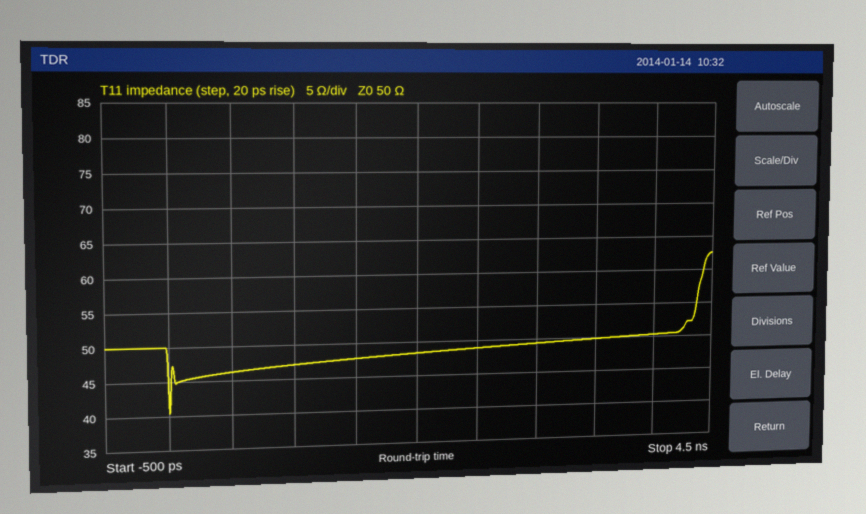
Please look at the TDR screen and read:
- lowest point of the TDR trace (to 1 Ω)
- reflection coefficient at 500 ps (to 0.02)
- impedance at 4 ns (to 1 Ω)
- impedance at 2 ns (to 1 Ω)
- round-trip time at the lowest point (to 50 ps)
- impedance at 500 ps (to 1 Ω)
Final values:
40 Ω
-0.04
50 Ω
48 Ω
0 ps
46 Ω
